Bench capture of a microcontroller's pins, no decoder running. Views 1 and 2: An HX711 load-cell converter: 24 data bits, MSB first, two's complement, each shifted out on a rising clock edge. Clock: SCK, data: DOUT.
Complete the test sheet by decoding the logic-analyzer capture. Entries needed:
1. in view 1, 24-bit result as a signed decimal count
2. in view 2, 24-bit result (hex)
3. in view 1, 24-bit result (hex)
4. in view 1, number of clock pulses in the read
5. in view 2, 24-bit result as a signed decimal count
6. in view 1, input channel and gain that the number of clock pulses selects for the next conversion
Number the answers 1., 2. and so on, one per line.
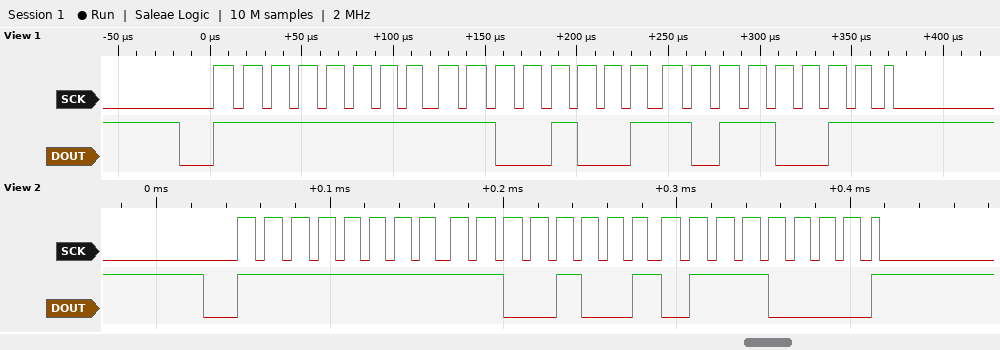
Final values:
1. -13901
2. 0xFFC970
3. 0xFFC9B3
4. 25
5. -13968
6. channel A, gain 128
